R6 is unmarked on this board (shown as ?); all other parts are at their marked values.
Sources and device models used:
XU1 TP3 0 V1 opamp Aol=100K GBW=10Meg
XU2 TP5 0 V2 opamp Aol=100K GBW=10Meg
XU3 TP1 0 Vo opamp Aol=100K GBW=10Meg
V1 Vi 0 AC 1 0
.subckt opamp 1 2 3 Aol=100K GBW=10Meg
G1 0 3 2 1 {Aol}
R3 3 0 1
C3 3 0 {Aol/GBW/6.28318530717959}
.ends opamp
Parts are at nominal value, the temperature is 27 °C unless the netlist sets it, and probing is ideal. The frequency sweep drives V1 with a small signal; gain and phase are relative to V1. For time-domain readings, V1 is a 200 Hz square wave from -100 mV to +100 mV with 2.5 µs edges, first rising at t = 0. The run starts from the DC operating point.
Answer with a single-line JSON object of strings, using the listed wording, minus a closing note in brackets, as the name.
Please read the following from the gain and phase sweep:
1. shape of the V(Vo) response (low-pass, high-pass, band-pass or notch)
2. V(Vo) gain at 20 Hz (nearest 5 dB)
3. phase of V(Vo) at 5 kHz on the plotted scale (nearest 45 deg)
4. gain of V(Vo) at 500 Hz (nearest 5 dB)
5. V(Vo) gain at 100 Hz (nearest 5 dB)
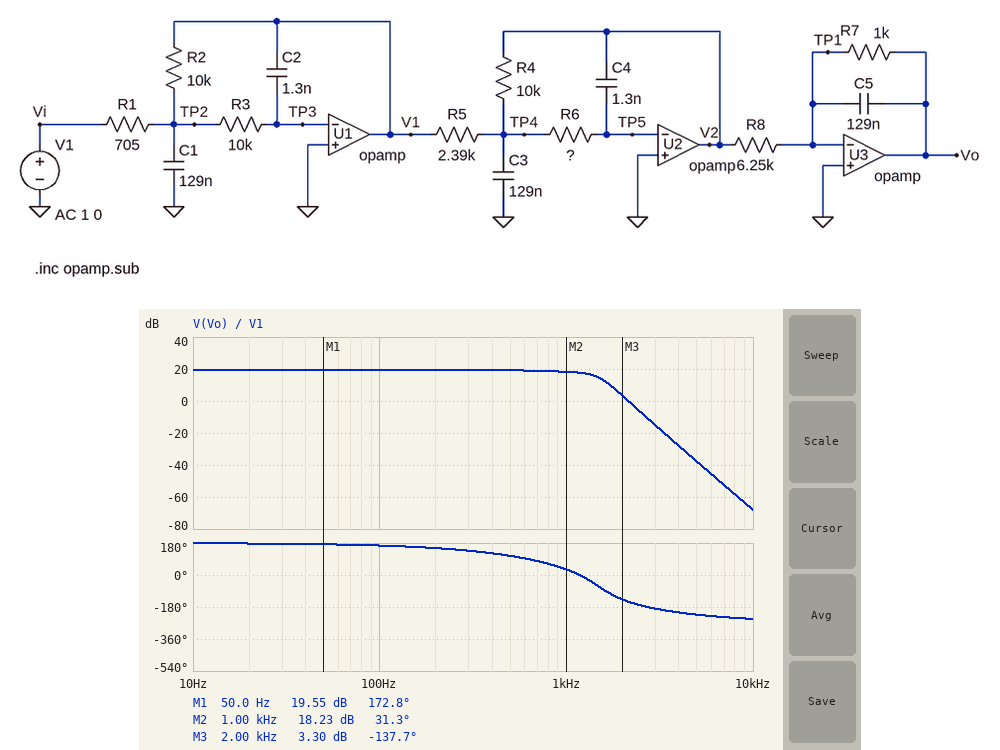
{"shape of the V(Vo) response": "low-pass", "V(Vo) gain at 20 Hz": "20 dB", "phase of V(Vo) at 5 kHz on the plotted scale": "-225 deg", "gain of V(Vo) at 500 Hz": "20 dB", "V(Vo) gain at 100 Hz": "20 dB"}
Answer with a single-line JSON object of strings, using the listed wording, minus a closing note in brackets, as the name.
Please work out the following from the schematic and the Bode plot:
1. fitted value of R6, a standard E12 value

{"fitted value of R6, a standard E12 value": "6.8 kΩ"}
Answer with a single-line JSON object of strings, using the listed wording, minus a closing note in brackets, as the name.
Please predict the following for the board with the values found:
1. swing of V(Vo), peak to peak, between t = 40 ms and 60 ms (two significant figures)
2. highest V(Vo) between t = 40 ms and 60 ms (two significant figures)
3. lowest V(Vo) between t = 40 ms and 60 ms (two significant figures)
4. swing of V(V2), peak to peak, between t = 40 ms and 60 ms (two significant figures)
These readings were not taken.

{"swing of V(Vo), peak to peak, between t = 40 ms and 60 ms": "2.2 V", "highest V(Vo) between t = 40 ms and 60 ms": "1.1 V", "lowest V(Vo) between t = 40 ms and 60 ms": "-1.1 V", "swing of V(V2), peak to peak, between t = 40 ms and 60 ms": "16 V"}
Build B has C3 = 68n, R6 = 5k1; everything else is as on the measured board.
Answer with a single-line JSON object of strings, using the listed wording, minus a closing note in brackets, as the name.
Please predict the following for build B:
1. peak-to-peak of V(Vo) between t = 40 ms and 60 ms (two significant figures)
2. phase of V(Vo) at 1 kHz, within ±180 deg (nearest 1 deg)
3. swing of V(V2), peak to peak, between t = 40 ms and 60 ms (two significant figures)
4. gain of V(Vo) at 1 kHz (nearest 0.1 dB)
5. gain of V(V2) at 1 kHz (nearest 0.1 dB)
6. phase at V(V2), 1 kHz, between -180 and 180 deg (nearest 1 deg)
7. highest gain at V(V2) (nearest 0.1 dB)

{"peak-to-peak of V(Vo) between t = 40 ms and 60 ms": "1.9 V", "phase of V(Vo) at 1 kHz, within ±180 deg": "45 deg", "swing of V(V2), peak to peak, between t = 40 ms and 60 ms": "12 V", "gain of V(Vo) at 1 kHz": "15.8 dB", "gain of V(V2) at 1 kHz": "33.9 dB", "phase at V(V2), 1 kHz, between -180 and 180 deg": "-96 deg", "highest gain at V(V2)": "35.5 dB"}
